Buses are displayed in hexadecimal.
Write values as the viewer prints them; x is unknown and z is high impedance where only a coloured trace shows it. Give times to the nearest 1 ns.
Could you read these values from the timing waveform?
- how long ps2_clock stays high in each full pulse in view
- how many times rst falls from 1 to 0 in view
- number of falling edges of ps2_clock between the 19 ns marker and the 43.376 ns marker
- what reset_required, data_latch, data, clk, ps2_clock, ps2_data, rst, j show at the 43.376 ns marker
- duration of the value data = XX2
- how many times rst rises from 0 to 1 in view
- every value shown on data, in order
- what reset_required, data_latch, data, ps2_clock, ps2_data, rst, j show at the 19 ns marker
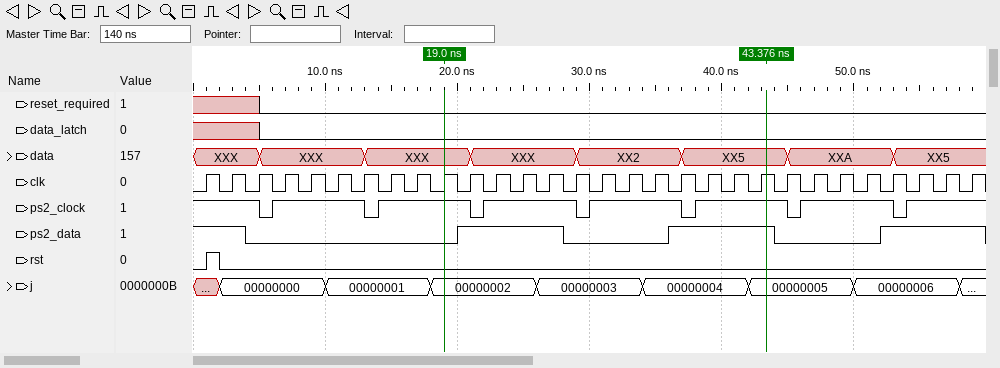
7 ns, 7 ns, 7 ns, 7 ns, 7 ns, 7 ns
1
3
reset_required=0, data_latch=0, data=XX5, clk=1, ps2_clock=1, ps2_data=1, rst=0, j=00000005
8 ns
1
XXX, XXX, XXX, XXX, XX2, XX5, XXA, XX5
reset_required=0, data_latch=0, data=XXX, ps2_clock=1, ps2_data=0, rst=0, j=00000002
